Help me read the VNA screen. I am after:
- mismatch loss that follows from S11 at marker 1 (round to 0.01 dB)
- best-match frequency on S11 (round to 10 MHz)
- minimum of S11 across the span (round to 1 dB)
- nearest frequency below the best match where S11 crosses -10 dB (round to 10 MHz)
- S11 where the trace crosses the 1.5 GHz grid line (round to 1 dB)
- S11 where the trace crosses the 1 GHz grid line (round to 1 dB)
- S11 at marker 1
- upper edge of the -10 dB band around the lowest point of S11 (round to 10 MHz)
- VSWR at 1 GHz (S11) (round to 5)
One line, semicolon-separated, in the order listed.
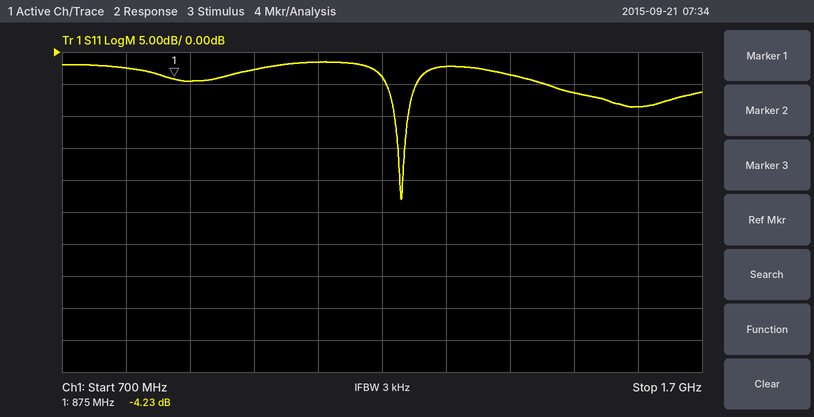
2.06 dB; 1.23 GHz; -23 dB; 1.22 GHz; -6 dB; -3 dB; -4.23 dB; 1.24 GHz; 5
